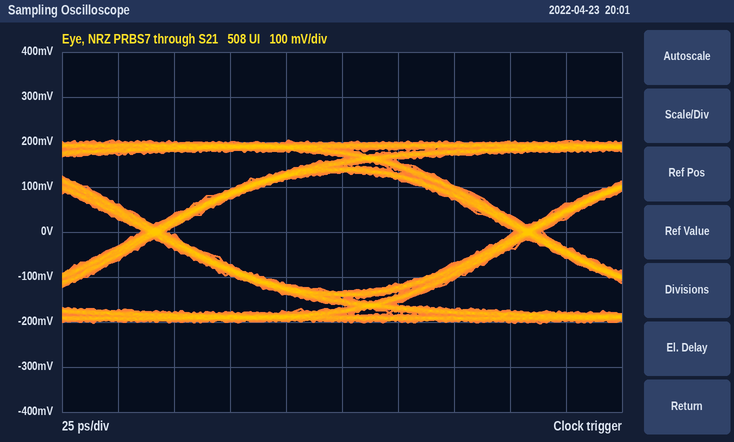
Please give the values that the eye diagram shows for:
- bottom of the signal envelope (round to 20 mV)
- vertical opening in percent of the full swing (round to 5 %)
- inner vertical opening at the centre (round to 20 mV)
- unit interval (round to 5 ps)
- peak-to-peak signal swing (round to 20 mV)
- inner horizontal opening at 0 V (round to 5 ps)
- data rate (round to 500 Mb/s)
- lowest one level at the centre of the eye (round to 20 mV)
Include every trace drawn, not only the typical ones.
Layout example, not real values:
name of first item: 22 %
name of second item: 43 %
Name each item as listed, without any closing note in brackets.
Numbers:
bottom of the signal envelope: -200 mV
vertical opening in percent of the full swing: 65 %
inner vertical opening at the centre: 260 mV
unit interval: 165 ps
peak-to-peak signal swing: 400 mV
inner horizontal opening at 0 V: 155 ps
data rate: 6.0 Gb/s
lowest one level at the centre of the eye: 140 mV
